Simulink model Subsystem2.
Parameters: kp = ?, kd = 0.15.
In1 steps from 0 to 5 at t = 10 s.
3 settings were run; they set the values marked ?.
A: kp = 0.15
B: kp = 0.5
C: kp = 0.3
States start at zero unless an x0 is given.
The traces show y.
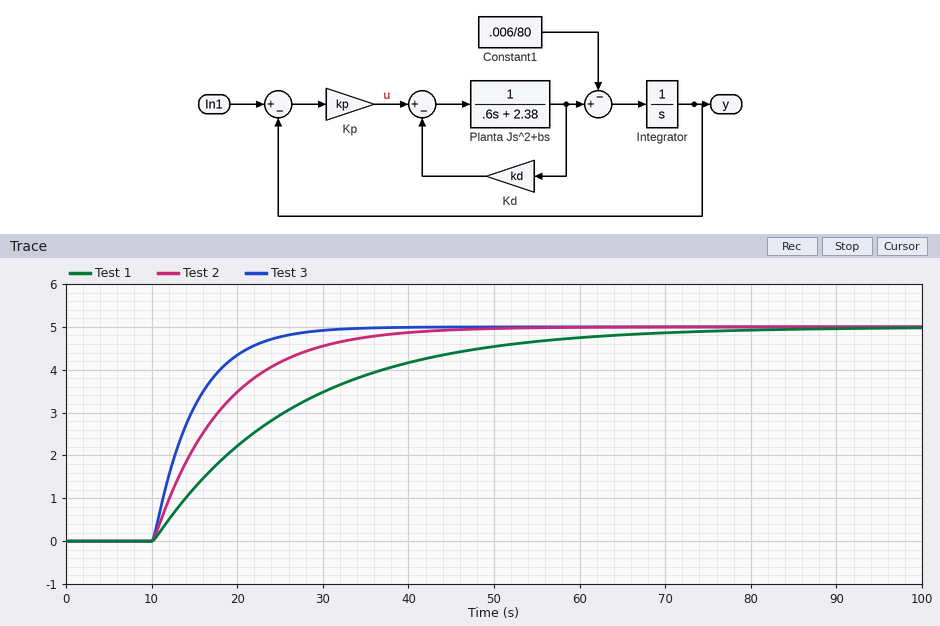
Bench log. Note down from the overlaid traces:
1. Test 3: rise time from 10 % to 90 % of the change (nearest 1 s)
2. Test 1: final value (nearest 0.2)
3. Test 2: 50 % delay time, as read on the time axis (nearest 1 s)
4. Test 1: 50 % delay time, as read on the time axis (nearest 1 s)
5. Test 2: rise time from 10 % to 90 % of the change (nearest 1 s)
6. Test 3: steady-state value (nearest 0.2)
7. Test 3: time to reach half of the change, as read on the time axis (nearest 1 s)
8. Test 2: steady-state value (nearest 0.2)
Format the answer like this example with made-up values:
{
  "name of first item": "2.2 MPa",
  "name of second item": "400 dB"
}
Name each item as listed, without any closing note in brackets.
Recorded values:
{
  "Test 3: rise time from 10 % to 90 % of the change": "11 s",
  "Test 1: final value": "5.0",
  "Test 2: 50 % delay time, as read on the time axis": "16 s",
  "Test 1: 50 % delay time, as read on the time axis": "22 s",
  "Test 2: rise time from 10 % to 90 % of the change": "18 s",
  "Test 3: steady-state value": "5.0",
  "Test 3: time to reach half of the change, as read on the time axis": "14 s",
  "Test 2: steady-state value": "5.0"
}
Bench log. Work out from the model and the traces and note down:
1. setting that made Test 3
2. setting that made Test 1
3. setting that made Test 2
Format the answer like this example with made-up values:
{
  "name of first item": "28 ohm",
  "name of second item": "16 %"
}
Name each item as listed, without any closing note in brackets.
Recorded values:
{
  "setting that made Test 3": "B",
  "setting that made Test 1": "A",
  "setting that made Test 2": "C"
}
